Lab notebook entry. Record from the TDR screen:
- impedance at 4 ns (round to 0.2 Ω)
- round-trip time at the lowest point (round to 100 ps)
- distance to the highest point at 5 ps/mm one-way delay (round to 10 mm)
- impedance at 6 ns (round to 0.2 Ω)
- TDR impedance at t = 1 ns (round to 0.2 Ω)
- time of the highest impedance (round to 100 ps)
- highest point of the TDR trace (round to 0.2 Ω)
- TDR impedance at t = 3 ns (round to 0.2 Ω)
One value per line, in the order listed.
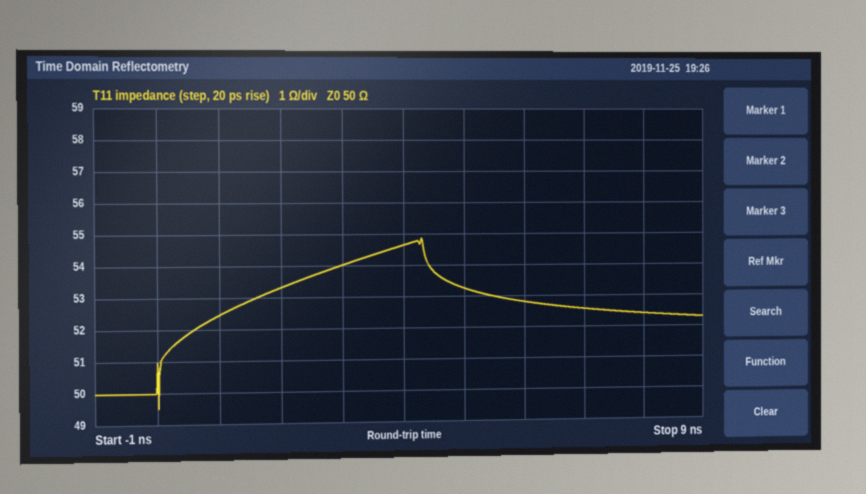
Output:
54.6 Ω
0.0 ns
430 mm
52.8 Ω
52.4 Ω
4.3 ns
54.8 Ω
54.0 Ω
